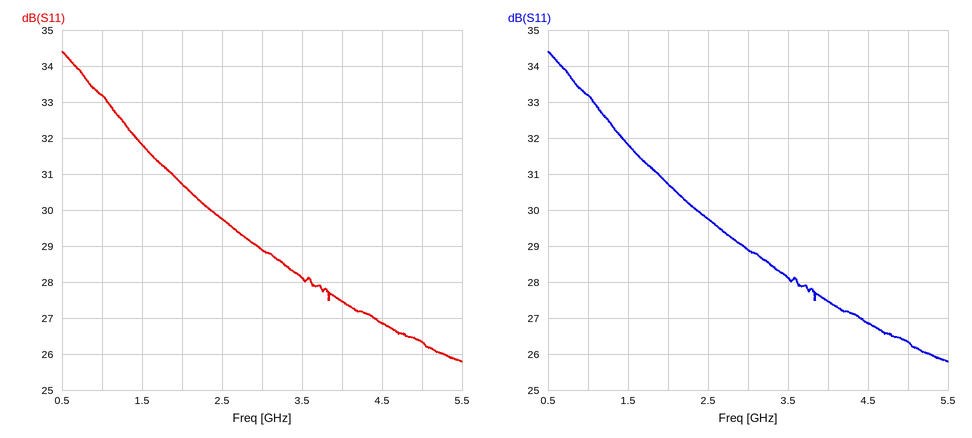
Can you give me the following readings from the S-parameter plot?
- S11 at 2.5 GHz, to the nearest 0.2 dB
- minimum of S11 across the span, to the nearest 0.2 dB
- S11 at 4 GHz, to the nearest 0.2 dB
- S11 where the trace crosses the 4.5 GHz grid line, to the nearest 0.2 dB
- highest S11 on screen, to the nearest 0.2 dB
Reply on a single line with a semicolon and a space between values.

29.8 dB; 25.8 dB; 27.4 dB; 26.8 dB; 34.4 dB
